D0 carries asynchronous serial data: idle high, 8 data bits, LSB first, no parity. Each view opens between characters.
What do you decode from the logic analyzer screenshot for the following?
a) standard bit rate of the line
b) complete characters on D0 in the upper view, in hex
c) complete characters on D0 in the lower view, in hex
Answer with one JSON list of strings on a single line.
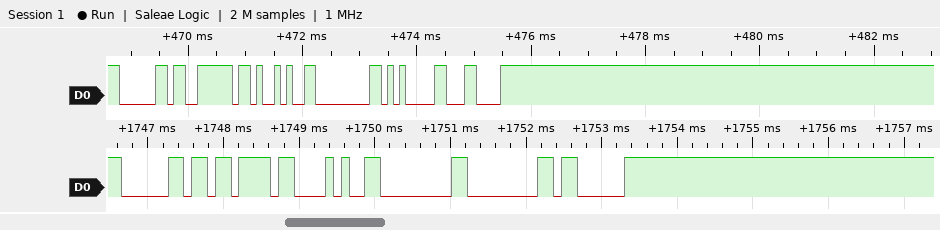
["9600 baud", "60, 7E, 29, 00, 05, 0C", "60, 7B, 28, 00, 00, 03"]
